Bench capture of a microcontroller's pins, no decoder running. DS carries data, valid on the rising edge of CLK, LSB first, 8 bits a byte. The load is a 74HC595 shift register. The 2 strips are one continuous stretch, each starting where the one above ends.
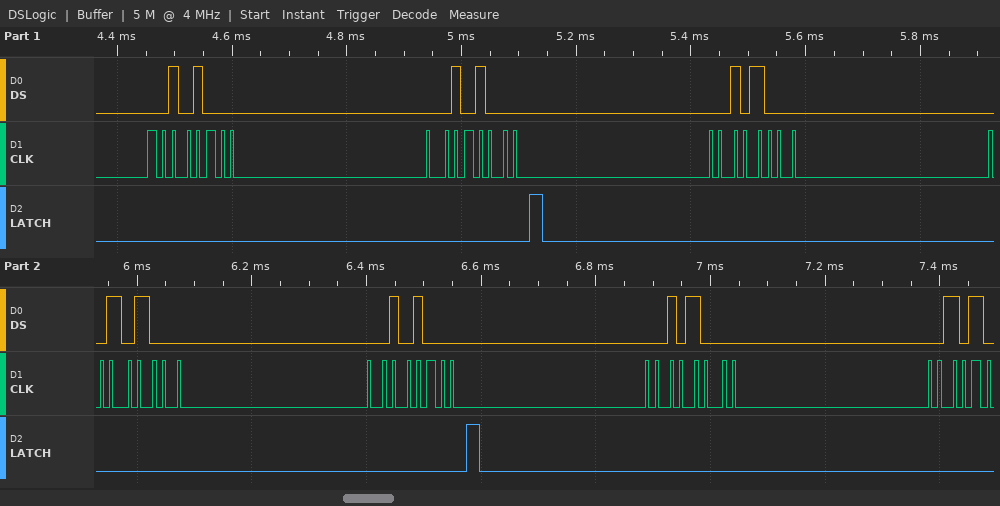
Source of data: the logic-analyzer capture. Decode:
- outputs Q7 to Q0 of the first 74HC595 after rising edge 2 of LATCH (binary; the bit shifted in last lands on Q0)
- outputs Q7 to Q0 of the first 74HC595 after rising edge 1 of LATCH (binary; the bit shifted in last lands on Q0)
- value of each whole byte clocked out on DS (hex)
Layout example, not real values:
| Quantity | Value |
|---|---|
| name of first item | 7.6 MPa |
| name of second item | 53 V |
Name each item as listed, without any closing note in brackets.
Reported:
| Quantity | Value |
|---|---|
| outputs Q7 to Q0 of the first 74HC595 after rising edge 2 of LATCH | 00101000 |
| outputs Q7 to Q0 of the first 74HC595 after rising edge 1 of LATCH | 00101000 |
| value of each whole byte clocked out on DS | 14 14 14 14 14 14 |
